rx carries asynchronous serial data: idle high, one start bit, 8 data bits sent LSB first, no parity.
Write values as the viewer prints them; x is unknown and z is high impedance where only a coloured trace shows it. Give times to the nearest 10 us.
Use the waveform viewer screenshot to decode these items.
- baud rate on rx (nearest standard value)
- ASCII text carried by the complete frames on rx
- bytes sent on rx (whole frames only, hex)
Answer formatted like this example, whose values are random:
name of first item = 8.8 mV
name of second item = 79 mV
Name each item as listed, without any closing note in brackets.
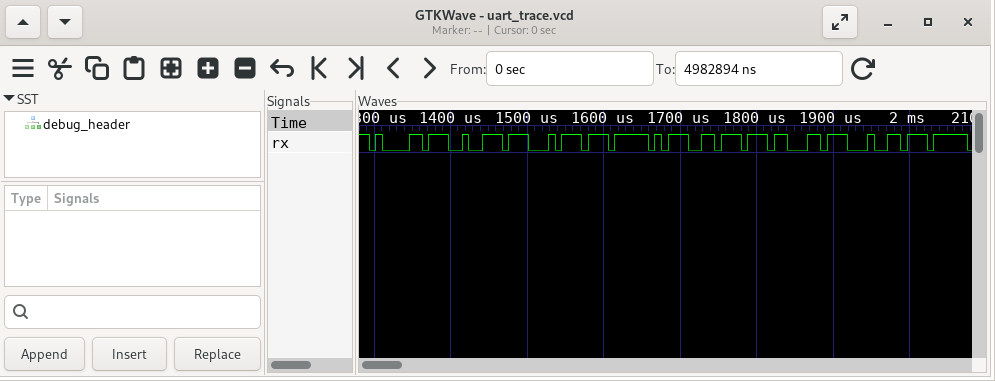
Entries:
baud rate on rx = 115200 baud
ASCII text carried by the complete frames on rx = "art_vcd"
bytes sent on rx = 61, 72, 74, 5F, 76, 63, 64
